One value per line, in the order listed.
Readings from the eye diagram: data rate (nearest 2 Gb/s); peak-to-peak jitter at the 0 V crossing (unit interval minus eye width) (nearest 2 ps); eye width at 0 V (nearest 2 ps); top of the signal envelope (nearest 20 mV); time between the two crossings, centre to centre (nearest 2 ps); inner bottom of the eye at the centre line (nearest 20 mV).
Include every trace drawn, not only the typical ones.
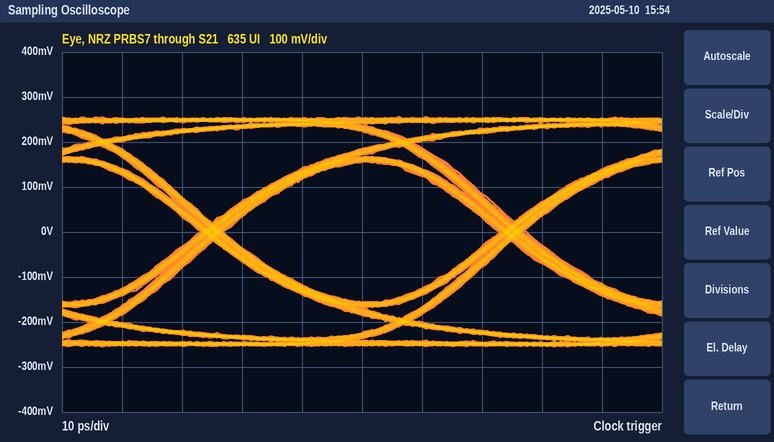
20 Gb/s
4 ps
46 ps
260 mV
50 ps
-160 mV
